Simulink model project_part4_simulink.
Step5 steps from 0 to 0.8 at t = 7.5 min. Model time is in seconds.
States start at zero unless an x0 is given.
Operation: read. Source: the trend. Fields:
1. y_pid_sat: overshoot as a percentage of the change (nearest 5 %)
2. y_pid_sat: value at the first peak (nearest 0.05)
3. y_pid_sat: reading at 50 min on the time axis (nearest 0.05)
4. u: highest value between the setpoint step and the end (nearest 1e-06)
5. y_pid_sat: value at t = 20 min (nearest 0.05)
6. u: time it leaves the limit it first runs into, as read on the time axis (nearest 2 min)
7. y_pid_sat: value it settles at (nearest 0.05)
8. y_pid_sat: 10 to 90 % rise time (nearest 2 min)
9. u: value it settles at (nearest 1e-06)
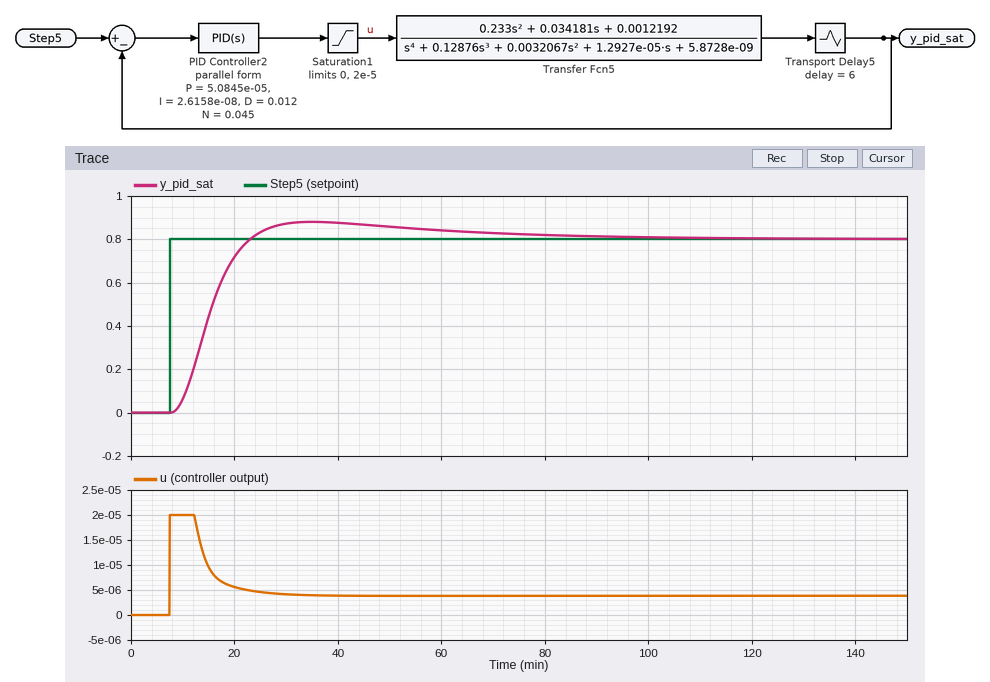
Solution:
10 %
0.90
0.85
0.000020
0.70
12 min
0.80
10 min
0.000004
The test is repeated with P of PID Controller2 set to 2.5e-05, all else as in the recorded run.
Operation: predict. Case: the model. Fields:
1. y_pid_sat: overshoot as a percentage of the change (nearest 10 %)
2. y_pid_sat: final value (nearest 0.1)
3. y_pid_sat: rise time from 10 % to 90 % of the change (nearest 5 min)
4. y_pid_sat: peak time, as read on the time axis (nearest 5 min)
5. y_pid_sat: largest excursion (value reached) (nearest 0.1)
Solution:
20 %
0.8
15 min
45 min
1.0
